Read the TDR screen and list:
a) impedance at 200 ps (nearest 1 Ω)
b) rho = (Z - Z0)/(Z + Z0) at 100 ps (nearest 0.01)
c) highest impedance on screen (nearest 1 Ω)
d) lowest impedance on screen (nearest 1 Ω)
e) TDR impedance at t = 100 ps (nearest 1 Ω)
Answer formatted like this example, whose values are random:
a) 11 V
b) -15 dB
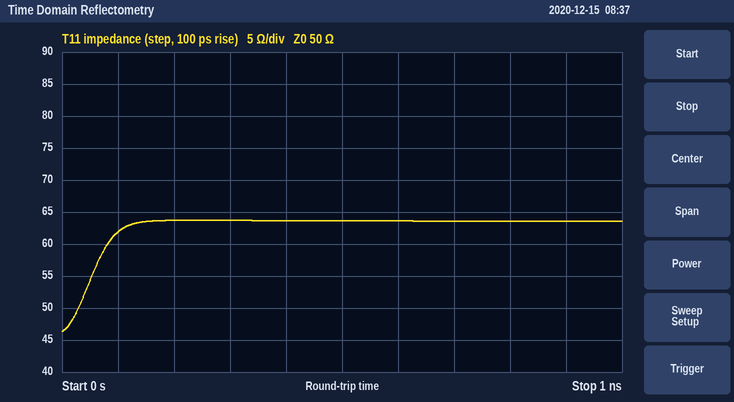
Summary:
a) 64 Ω
b) +0.11
c) 64 Ω
d) 46 Ω
e) 62 Ω
